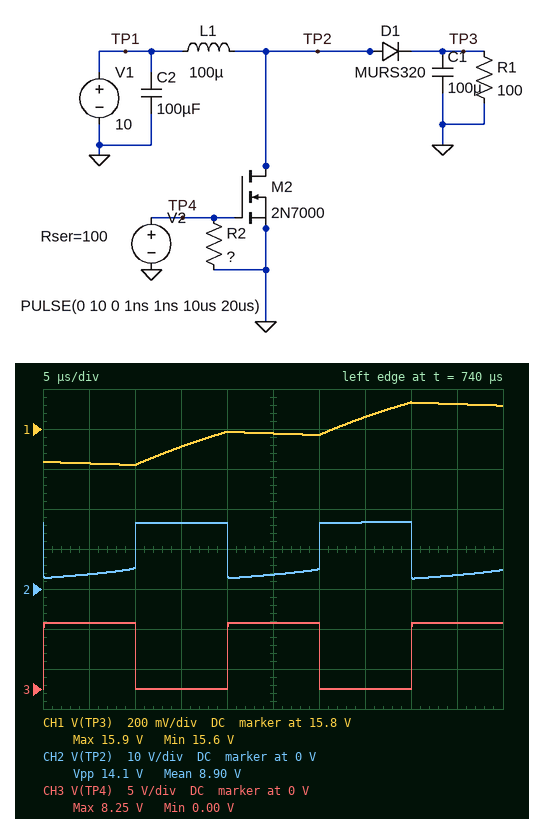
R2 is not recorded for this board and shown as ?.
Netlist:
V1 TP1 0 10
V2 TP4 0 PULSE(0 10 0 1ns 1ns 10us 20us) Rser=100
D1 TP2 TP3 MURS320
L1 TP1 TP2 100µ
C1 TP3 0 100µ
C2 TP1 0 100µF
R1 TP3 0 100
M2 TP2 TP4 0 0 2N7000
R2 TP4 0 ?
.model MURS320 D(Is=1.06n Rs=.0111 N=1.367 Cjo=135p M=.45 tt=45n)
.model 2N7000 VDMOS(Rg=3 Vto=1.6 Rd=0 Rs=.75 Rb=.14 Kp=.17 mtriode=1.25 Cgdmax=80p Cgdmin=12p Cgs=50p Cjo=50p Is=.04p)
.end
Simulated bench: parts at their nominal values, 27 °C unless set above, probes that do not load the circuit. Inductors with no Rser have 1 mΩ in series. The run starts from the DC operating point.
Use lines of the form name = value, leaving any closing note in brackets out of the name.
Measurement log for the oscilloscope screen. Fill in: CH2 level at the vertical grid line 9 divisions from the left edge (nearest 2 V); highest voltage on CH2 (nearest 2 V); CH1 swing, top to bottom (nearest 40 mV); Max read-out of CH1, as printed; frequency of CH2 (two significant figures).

CH2 level at the vertical grid line 9 divisions from the left edge = 4 V
highest voltage on CH2 = 16 V
CH1 swing, top to bottom = 320 mV
Max read-out of CH1, as printed = 15.9 V
frequency of CH2 = 50 kHz
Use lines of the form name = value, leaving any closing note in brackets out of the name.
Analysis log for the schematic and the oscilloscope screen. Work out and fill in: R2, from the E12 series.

R2, from the E12 series = 470 Ω
